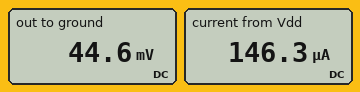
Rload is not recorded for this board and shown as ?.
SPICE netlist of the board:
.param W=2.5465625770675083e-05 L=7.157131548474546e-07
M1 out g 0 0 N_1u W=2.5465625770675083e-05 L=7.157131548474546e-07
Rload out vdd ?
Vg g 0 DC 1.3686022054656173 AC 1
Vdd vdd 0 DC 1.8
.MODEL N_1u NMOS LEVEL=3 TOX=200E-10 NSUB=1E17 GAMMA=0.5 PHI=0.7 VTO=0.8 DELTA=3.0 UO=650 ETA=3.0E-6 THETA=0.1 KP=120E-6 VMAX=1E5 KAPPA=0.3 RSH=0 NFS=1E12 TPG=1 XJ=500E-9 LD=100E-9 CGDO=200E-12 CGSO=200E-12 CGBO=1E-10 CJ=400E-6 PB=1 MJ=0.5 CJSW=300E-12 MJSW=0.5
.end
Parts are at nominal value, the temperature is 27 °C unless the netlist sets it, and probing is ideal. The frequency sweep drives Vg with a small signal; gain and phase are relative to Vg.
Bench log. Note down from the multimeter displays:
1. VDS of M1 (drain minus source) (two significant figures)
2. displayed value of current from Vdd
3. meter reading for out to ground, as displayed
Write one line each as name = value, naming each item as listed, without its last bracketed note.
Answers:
VDS of M1 (drain minus source) = 45 mV
displayed value of current from Vdd = 146.3 µA
meter reading for out to ground, as displayed = 44.6 mV
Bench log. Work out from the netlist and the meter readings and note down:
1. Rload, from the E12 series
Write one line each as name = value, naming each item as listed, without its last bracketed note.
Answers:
Rload, from the E12 series = 12 kΩ
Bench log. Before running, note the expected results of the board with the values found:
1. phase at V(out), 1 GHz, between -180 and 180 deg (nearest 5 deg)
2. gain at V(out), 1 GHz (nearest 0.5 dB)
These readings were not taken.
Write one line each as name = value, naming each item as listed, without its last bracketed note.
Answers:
phase at V(out), 1 GHz, between -180 and 180 deg = 155 deg
gain at V(out), 1 GHz = -22.0 dB
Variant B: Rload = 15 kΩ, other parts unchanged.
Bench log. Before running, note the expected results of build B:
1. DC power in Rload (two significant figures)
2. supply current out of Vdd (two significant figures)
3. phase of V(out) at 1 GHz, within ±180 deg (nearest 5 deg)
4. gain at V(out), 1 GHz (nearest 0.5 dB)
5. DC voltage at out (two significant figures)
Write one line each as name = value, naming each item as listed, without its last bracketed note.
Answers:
DC power in Rload = 210 µW
supply current out of Vdd = 120 µA
phase of V(out) at 1 GHz, within ±180 deg = 150 deg
gain at V(out), 1 GHz = -24.0 dB
DC voltage at out = 35 mV
